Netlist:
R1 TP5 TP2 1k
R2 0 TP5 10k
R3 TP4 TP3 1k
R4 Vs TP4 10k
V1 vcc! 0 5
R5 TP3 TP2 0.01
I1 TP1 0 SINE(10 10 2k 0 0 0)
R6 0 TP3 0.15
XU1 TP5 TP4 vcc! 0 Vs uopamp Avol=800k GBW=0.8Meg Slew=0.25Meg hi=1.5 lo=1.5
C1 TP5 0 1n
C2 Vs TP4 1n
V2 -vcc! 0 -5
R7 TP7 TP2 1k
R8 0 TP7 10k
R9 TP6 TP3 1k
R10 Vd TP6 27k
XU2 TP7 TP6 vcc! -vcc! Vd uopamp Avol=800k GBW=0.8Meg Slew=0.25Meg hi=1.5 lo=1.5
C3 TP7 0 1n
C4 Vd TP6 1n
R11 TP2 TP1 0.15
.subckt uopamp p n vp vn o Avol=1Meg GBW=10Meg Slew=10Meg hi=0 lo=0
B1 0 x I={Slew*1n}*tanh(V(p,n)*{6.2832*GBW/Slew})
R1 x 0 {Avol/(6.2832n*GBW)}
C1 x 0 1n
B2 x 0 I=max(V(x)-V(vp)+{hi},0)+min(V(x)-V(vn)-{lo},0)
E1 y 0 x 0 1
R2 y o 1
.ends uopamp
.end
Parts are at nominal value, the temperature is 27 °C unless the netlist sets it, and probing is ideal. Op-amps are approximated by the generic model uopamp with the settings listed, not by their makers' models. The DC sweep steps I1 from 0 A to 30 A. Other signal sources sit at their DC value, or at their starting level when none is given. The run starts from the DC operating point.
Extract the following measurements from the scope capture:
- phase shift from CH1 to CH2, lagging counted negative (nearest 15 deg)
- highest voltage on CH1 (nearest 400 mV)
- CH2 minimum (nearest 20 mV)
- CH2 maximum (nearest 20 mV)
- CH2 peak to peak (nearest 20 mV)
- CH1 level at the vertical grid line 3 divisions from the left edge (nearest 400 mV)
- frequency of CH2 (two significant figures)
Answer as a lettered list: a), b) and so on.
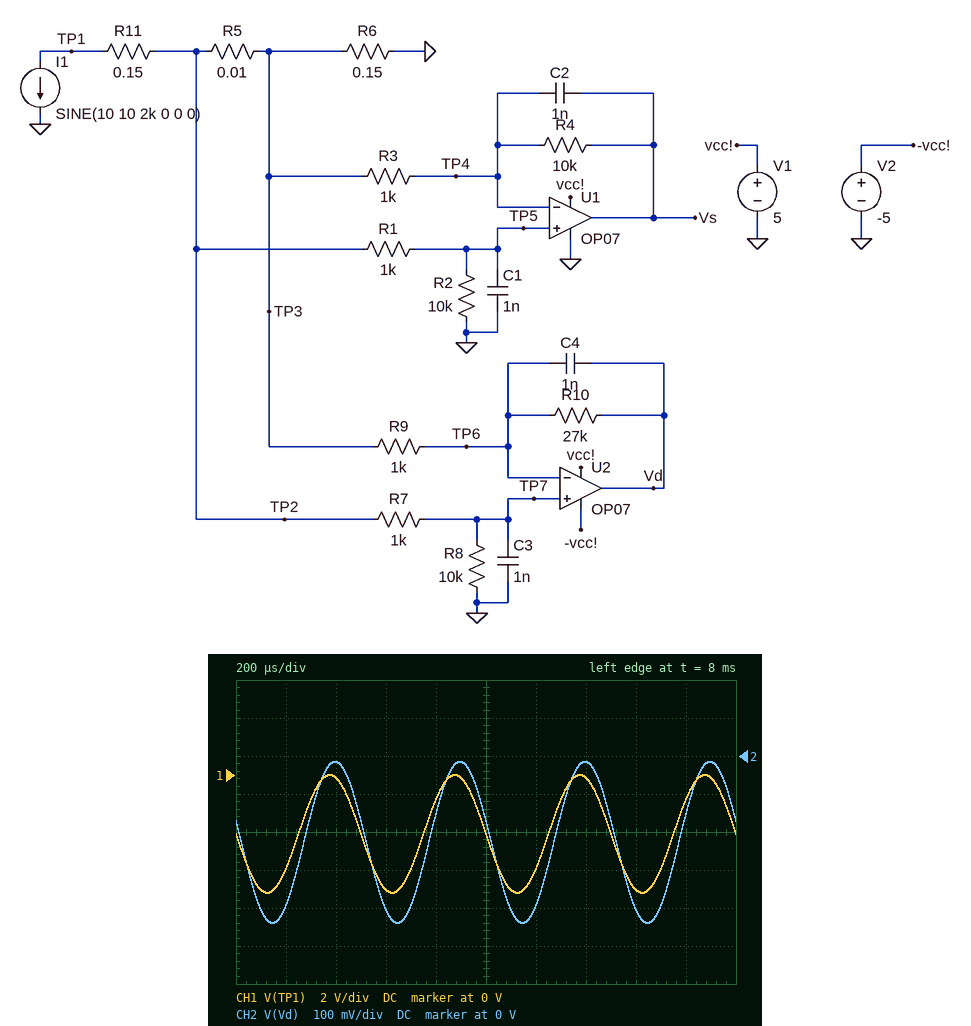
a) -15 deg
b) 0 V
c) -440 mV
d) -20 mV
e) 420 mV
f) -6.0 V
g) 2.0 kHz
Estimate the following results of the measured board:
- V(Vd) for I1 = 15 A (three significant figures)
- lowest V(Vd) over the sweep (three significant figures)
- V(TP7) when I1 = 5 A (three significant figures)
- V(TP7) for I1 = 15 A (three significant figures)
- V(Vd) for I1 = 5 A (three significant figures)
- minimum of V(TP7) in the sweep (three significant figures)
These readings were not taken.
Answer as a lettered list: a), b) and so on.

a) -341 mV
b) -682 mV
c) -727 mV
d) -2.18 V
e) -114 mV
f) -4.36 V
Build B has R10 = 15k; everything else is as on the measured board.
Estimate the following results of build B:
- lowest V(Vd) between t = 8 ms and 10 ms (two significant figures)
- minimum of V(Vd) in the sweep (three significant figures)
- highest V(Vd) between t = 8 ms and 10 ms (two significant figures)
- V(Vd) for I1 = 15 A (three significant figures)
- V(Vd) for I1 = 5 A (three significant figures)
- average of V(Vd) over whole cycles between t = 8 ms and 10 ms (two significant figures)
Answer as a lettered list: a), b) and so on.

a) -1.5 V
b) -2.32 V
c) -19 mV
d) -1.16 V
e) -386 mV
f) -770 mV
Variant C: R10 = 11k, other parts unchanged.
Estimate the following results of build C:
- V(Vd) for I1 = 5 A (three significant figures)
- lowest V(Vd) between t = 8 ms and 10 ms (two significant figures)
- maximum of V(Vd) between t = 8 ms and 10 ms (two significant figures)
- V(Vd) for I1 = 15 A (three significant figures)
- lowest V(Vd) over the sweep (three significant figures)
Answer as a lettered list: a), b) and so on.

a) -477 mV
b) -1.9 V
c) -13 mV
d) -1.43 V
e) -2.86 V
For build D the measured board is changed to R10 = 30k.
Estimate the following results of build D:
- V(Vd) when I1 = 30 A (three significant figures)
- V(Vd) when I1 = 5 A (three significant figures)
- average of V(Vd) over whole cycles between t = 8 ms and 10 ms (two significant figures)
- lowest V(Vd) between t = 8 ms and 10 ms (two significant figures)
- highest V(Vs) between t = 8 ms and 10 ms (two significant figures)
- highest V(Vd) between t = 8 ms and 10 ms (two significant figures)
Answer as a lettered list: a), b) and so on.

a) -273 mV
b) -45.5 mV
c) -91 mV
d) -180 mV
e) 1.5 V
f) -2.4 mV
